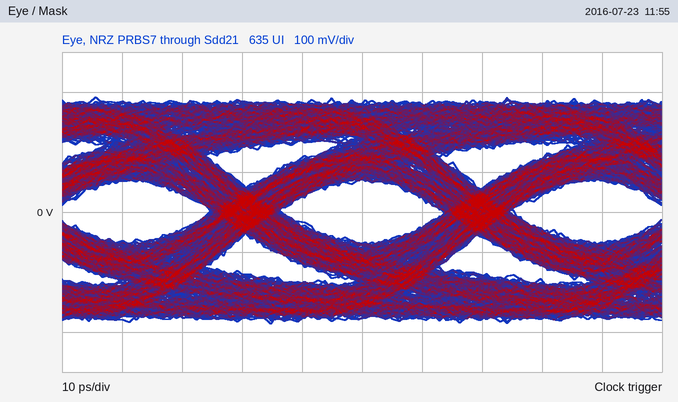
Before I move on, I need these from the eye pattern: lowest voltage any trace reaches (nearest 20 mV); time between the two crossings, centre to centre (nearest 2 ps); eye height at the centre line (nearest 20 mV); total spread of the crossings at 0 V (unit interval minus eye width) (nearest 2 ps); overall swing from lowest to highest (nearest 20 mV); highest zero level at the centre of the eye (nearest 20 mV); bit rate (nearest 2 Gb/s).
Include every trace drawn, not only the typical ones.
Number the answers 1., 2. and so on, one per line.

1. -280 mV
2. 38 ps
3. 160 mV
4. 12 ps
5. 560 mV
6. -80 mV
7. 26 Gb/s
